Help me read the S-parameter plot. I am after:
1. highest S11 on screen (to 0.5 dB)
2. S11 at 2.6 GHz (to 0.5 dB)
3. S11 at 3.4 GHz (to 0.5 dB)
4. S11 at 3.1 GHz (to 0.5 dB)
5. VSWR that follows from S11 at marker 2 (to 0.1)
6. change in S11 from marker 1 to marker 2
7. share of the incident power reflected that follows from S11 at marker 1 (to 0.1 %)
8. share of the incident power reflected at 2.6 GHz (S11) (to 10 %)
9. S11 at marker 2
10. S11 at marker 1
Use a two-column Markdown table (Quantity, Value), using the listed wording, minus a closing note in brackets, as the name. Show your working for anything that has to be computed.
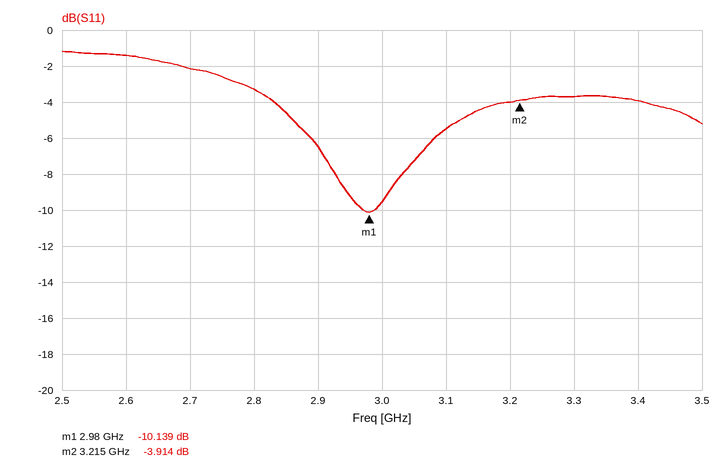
| Quantity | Value |
|---|---|
| highest S11 on screen | -1.0 dB |
| S11 at 2.6 GHz | -1.5 dB |
| S11 at 3.4 GHz | -4.0 dB |
| S11 at 3.1 GHz | -5.5 dB |
| VSWR that follows from S11 at marker 2 | (1 + 0.6372)/(1 − 0.6372) ≈ 4.5 |
| change in S11 from marker 1 to marker 2 | -3.914 − (-10.139) = 6.225 dB |
| share of the incident power reflected that follows from S11 at marker 1 | 10^(-10.139/10) ≈ 9.7 % |
| share of the incident power reflected at 2.6 GHz (S11) | 10^(-1.5/10) ≈ 70.8 %, so 70 % to the nearest 10 % |
| S11 at marker 2 | -3.914 dB |
| S11 at marker 1 | -10.139 dB |
